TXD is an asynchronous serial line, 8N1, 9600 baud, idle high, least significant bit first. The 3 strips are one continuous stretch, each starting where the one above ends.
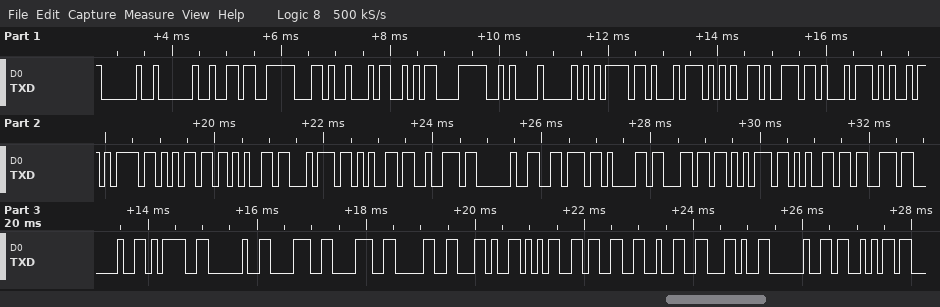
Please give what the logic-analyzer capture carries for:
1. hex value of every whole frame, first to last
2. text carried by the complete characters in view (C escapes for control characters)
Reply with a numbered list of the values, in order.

1. 20 20 36 2C 34 0D 0A 50 6F 74 65 6E 74 69 6F 6D 65 74 65 72 20 76 61 6C 75 65 73 20 3D 20 38 38 30 2C 35 33 32 2C 20 53
2. "  6,4\r\nPotentiometer values = 880,532, S"
